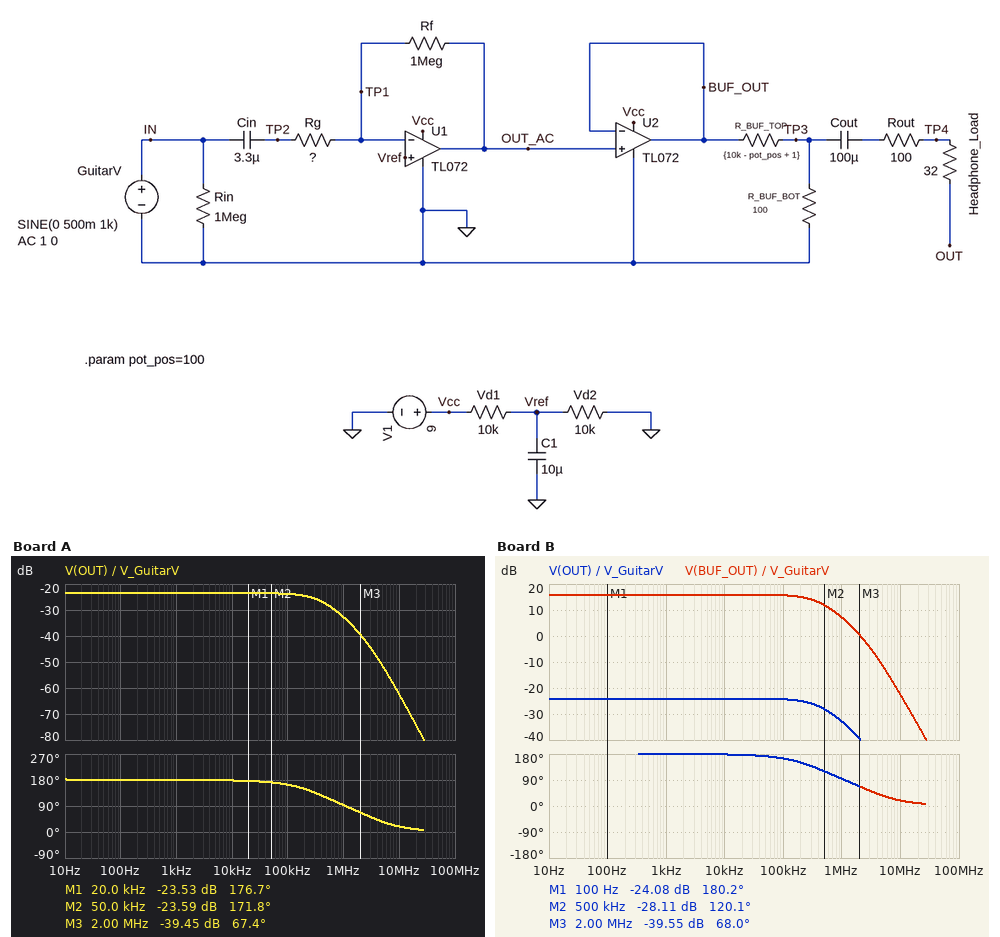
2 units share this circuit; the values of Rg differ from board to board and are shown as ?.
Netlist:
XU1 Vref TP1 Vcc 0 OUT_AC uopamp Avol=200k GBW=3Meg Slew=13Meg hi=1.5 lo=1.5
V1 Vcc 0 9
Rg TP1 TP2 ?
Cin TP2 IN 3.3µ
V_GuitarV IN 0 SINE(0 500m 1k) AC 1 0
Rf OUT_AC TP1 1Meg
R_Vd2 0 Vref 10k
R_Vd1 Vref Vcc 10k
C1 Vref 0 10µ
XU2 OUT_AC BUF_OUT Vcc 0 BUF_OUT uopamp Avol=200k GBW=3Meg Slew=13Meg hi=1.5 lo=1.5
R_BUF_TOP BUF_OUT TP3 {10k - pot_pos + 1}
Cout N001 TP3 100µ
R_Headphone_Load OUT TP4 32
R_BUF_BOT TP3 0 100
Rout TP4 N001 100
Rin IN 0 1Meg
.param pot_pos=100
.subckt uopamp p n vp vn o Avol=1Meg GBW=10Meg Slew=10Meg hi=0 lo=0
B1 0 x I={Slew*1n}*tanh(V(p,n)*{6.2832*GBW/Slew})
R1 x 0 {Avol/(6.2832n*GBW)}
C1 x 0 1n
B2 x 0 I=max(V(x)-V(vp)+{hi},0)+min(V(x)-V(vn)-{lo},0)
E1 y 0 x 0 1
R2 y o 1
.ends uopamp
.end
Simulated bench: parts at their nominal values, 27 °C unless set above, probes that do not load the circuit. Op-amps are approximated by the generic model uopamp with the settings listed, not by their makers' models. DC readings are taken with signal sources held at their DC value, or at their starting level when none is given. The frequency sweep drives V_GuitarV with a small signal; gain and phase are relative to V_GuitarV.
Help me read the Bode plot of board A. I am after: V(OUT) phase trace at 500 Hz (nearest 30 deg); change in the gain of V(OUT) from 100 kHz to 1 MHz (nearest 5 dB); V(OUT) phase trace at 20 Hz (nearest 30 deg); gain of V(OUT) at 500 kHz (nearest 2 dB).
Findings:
180 deg
-10 dB
180 deg
-28 dB
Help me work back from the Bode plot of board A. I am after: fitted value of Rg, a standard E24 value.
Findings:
150 kΩ
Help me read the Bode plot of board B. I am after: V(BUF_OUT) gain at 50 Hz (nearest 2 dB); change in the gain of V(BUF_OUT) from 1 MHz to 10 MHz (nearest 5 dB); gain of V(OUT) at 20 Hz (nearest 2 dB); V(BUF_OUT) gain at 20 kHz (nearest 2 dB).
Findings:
16 dB
-30 dB
-24 dB
16 dB
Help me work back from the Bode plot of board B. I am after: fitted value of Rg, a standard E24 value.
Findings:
160 kΩ
